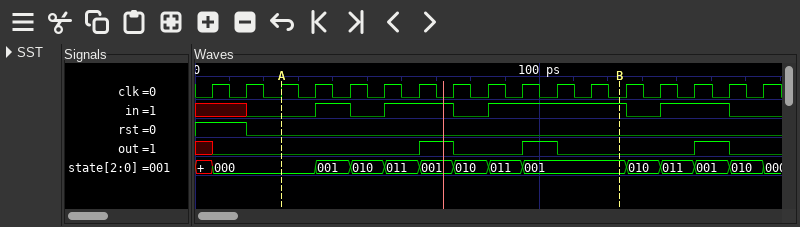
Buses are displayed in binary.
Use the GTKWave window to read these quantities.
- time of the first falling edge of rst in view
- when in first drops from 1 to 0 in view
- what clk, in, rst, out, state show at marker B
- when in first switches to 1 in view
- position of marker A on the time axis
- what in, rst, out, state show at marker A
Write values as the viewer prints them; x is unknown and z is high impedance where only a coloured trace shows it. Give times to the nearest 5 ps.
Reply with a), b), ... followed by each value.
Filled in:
a) 15 ps
b) 45 ps
c) clk=0, in=1, rst=0, out=0, state=001
d) 35 ps
e) 25 ps
f) in=0, rst=0, out=0, state=000
